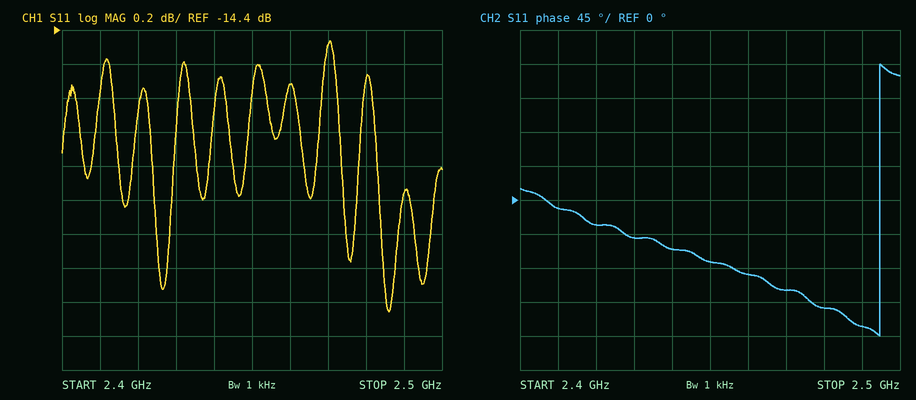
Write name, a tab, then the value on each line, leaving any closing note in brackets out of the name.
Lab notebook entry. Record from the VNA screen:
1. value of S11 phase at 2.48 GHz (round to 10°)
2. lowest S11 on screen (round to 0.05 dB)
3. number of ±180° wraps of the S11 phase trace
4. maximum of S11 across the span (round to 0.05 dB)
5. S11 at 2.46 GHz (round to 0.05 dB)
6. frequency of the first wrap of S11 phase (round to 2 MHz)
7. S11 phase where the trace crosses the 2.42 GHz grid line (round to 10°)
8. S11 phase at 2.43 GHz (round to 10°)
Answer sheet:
value of S11 phase at 2.48 GHz	-140°
lowest S11 on screen	-16.05 dB
number of ±180° wraps of the S11 phase trace	1
maximum of S11 across the span	-14.45 dB
S11 at 2.46 GHz	-14.70 dB
frequency of the first wrap of S11 phase	2.494 GHz
S11 phase where the trace crosses the 2.42 GHz grid line	-30°
S11 phase at 2.43 GHz	-50°
